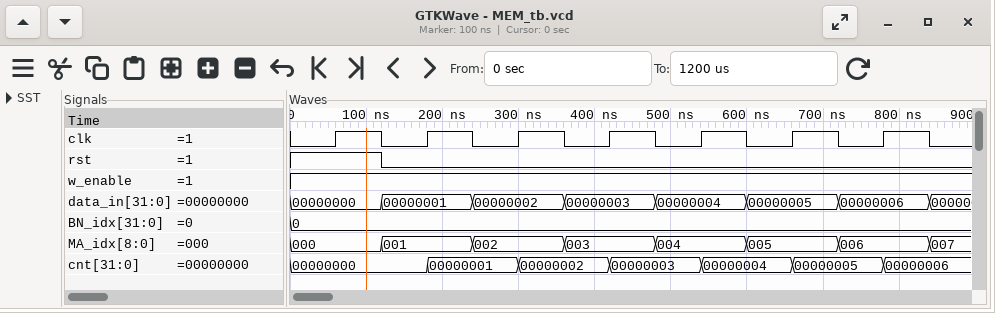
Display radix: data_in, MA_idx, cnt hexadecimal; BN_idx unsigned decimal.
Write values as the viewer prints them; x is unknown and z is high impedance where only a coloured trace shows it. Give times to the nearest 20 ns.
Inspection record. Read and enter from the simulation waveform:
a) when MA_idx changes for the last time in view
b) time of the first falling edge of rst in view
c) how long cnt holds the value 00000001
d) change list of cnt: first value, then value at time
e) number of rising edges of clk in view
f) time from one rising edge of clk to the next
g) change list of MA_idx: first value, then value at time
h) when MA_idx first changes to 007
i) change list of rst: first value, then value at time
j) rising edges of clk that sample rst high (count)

840 ns
120 ns
120 ns
00000000, 00000001 at 180 ns, 00000002 at 300 ns, 00000003 at 420 ns, 00000004 at 540 ns, 00000005 at 660 ns, 00000006 at 780 ns
7
120 ns
000, 001 at 120 ns, 002 at 240 ns, 003 at 360 ns, 004 at 480 ns, 005 at 600 ns, 006 at 720 ns, 007 at 840 ns
840 ns
1, 0 at 120 ns
1
